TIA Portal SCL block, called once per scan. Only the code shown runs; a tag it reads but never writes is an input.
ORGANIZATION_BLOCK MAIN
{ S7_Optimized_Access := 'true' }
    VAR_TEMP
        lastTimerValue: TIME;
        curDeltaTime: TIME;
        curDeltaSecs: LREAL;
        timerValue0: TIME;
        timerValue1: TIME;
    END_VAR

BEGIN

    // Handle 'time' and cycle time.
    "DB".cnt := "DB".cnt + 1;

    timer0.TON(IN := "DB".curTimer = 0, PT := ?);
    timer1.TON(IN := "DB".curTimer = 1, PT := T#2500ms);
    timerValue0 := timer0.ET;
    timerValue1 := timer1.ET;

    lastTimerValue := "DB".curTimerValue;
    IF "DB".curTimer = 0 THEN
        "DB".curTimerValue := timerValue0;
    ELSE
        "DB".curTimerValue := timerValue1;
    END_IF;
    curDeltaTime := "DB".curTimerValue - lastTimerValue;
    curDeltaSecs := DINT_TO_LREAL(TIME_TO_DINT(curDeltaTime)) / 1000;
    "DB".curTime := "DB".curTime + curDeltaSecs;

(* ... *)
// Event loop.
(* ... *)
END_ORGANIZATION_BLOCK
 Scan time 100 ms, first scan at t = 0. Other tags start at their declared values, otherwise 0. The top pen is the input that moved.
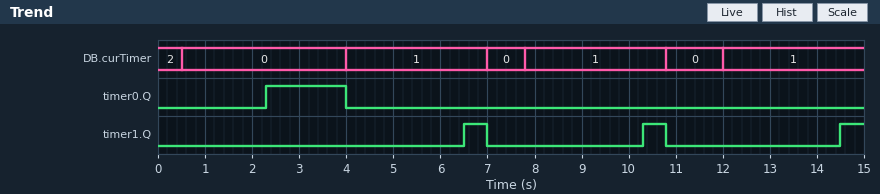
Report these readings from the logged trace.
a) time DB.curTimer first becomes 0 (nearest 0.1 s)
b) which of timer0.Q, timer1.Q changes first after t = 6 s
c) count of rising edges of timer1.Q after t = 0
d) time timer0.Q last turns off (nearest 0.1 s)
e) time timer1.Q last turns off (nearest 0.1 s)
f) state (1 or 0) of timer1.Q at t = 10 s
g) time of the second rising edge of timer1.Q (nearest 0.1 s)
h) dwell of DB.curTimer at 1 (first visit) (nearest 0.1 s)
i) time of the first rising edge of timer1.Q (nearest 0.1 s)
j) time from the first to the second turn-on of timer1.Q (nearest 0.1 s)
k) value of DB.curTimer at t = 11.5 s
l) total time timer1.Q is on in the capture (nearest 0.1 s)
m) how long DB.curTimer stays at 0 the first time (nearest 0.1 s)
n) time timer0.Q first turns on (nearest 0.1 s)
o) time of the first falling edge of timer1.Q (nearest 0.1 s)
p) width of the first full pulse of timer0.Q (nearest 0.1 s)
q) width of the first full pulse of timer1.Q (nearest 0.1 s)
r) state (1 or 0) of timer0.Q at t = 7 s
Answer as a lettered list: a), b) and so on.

a) 0.5 s
b) timer1.Q
c) 3
d) 4.0 s
e) 10.8 s
f) 0
g) 10.3 s
h) 3.0 s
i) 6.5 s
j) 3.8 s
k) 0
l) 1.5 s
m) 3.5 s
n) 2.3 s
o) 7.0 s
p) 1.7 s
q) 0.5 s
r) 0
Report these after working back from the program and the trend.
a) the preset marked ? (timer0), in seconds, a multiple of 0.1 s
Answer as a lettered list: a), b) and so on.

a) 1.8 s
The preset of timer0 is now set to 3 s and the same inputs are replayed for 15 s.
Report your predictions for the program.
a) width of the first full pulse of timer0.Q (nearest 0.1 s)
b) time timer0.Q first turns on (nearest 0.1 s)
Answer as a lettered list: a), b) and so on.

a) 0.5 s
b) 3.5 s
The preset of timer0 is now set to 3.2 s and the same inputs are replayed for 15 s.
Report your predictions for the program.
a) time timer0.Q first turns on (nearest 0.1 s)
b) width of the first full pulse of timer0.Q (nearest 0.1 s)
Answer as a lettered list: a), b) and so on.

a) 3.7 s
b) 0.3 s
